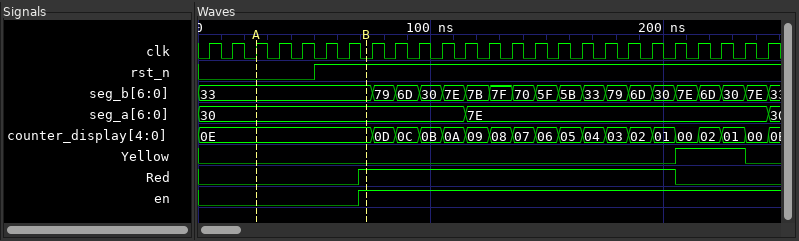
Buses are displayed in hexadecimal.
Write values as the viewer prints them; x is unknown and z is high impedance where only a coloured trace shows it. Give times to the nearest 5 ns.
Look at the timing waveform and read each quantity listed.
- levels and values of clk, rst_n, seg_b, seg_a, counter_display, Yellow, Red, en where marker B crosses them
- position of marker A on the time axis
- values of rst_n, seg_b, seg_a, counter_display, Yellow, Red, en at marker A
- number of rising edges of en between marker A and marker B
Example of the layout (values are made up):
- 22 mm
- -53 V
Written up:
- clk=0, rst_n=1, seg_b=33, seg_a=30, counter_display=0E, Yellow=0, Red=1, en=1
- 25 ns
- rst_n=0, seg_b=33, seg_a=30, counter_display=0E, Yellow=0, Red=0, en=0
- 1
